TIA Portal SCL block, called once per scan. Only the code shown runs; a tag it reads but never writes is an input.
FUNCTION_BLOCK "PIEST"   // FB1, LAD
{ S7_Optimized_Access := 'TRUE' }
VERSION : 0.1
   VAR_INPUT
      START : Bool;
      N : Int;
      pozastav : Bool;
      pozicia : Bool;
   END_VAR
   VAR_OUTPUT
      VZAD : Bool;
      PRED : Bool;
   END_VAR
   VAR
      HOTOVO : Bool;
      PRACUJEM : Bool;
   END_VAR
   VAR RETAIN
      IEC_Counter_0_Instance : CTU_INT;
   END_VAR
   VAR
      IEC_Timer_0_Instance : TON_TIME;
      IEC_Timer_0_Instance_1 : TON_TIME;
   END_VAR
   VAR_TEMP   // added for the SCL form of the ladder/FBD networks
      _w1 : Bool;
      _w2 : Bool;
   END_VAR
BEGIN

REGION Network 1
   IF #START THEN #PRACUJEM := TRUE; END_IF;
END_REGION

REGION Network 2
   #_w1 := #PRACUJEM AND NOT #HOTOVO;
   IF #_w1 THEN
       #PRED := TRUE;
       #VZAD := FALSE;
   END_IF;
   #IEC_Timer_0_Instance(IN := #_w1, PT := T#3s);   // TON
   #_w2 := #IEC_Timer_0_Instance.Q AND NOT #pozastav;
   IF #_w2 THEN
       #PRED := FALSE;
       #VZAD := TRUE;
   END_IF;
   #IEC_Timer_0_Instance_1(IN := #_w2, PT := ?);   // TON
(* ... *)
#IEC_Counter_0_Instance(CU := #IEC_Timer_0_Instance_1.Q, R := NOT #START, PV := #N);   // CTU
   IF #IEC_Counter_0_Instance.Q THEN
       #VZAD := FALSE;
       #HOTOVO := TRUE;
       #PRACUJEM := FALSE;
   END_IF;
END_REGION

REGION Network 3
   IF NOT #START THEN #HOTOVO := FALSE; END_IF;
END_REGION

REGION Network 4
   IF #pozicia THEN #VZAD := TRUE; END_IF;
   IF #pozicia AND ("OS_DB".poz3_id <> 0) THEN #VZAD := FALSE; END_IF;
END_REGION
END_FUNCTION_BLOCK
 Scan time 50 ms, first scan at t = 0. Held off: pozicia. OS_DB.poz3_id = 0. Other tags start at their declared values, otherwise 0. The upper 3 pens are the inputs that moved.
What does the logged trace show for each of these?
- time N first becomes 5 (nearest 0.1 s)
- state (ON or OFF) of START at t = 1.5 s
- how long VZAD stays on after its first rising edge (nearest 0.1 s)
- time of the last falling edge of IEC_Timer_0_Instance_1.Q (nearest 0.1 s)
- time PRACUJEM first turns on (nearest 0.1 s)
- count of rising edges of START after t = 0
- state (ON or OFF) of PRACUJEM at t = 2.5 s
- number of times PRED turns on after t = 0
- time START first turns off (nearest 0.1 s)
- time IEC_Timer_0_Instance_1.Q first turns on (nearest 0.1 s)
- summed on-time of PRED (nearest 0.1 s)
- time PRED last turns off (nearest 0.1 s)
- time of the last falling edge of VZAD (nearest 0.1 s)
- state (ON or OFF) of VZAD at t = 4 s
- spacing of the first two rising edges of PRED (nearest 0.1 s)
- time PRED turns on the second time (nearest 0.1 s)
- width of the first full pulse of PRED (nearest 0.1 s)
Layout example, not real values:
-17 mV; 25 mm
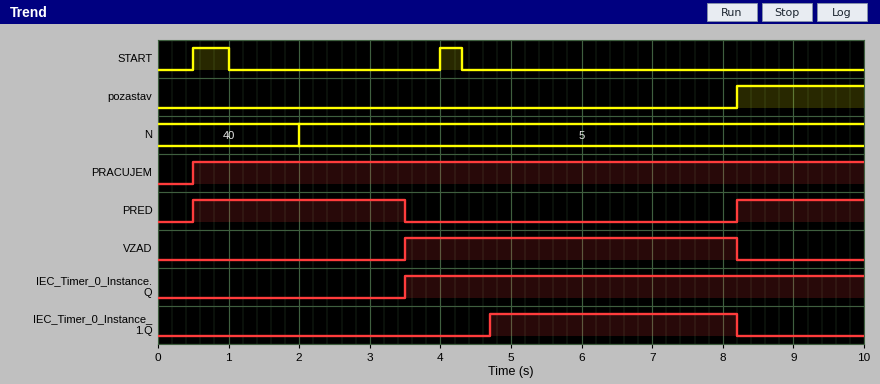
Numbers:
2.0 s; OFF; 4.7 s; 8.2 s; 0.5 s; 2; ON; 2; 1.0 s; 4.7 s; 4.8 s; 3.5 s; 8.2 s; ON; 7.7 s; 8.2 s; 3.0 s
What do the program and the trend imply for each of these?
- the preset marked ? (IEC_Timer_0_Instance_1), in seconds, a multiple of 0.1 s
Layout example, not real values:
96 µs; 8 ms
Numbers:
1.2 s
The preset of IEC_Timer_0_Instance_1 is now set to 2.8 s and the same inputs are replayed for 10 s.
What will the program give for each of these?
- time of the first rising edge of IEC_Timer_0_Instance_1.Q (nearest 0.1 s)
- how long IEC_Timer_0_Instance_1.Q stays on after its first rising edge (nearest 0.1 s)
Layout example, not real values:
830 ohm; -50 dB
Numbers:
6.3 s; 1.9 s
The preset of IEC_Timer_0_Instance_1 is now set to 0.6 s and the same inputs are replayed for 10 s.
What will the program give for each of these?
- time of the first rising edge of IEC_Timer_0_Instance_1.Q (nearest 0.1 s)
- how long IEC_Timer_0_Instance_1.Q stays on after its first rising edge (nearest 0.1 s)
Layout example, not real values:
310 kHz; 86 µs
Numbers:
4.1 s; 4.1 s
